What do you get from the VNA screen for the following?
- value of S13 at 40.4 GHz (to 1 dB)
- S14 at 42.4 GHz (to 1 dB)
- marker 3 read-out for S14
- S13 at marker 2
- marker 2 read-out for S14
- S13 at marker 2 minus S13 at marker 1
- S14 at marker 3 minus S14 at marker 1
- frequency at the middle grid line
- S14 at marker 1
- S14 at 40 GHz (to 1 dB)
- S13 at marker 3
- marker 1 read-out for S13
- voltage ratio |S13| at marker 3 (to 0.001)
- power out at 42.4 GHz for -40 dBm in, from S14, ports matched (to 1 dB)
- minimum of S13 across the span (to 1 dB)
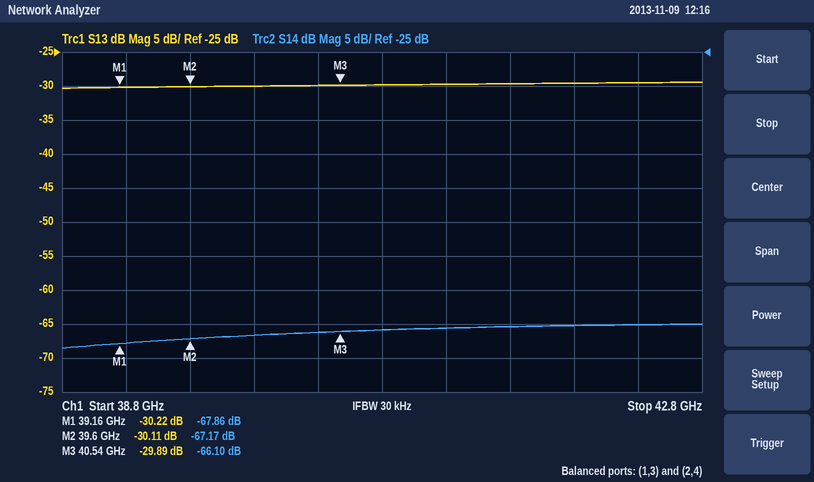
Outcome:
-30 dB
-65 dB
-66.10 dB
-30.11 dB
-67.17 dB
0.11 dB
1.76 dB
40.8 GHz
-67.86 dB
-67 dB
-29.89 dB
-30.22 dB
0.032
-105 dBm
-30 dB
